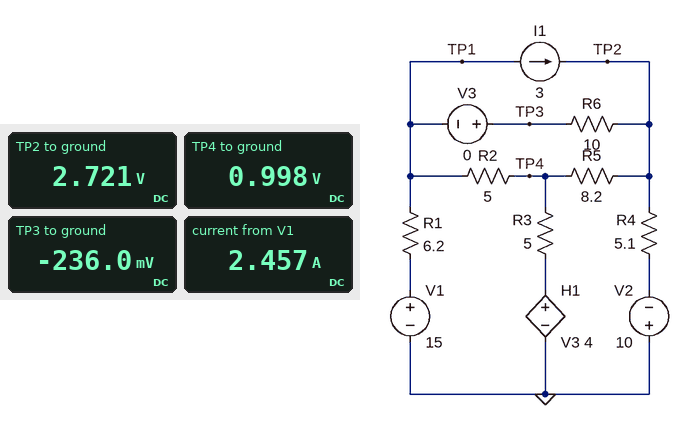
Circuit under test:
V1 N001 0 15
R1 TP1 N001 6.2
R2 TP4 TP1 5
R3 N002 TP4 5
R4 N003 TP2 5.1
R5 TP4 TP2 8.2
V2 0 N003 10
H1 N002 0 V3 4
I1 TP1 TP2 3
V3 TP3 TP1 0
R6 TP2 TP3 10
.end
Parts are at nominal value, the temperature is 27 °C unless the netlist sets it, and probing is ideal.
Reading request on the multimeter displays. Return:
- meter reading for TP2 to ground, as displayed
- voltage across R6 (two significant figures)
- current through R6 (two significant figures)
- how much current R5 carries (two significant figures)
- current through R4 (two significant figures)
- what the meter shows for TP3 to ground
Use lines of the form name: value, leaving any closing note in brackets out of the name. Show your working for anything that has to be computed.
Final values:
meter reading for TP2 to ground, as displayed: 2.721 V
voltage across R6: 2.721 V - (-236 mV) = 3.0 V
current through R6: (2.721 V - (-236 mV)) / 10 Ω = 300 mA
how much current R5 carries: (2.721 V - 998 mV) / 8.2 Ω = 210 mA
current through R4: (2.721 V - (-10 V)) / 5.1 Ω = 2.5 A
what the meter shows for TP3 to ground: -236.0 mV
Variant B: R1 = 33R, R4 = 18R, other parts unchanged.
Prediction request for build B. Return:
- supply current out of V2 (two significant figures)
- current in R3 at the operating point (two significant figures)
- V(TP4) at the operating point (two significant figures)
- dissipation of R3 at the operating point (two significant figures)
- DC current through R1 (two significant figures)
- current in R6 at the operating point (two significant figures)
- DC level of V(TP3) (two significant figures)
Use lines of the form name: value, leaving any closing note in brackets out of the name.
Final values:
supply current out of V2: 1.0 A
current in R3 at the operating point: 470 mA
V(TP4) at the operating point: 2.5 V
dissipation of R3 at the operating point: 1.1 W
DC current through R1: 560 mA
current in R6 at the operating point: 1.2 A
DC level of V(TP3): -3.6 V
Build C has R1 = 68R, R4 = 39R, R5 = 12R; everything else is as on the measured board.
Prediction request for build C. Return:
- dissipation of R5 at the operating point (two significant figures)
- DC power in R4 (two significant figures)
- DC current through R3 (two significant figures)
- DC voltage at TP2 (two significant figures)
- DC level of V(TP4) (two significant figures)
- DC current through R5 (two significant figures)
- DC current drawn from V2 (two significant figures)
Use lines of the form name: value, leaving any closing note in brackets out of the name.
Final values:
dissipation of R5 at the operating point: 7.9 W
DC power in R4: 15 W
DC current through R3: 380 mA
DC voltage at TP2: 14 V
DC level of V(TP4): 4.4 V
DC current through R5: 810 mA
DC current drawn from V2: 620 mA
